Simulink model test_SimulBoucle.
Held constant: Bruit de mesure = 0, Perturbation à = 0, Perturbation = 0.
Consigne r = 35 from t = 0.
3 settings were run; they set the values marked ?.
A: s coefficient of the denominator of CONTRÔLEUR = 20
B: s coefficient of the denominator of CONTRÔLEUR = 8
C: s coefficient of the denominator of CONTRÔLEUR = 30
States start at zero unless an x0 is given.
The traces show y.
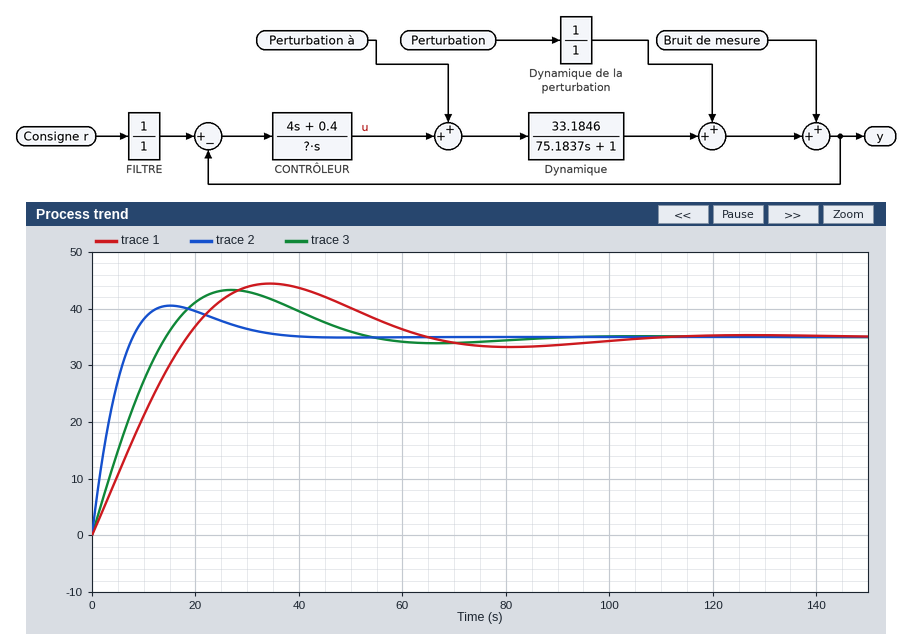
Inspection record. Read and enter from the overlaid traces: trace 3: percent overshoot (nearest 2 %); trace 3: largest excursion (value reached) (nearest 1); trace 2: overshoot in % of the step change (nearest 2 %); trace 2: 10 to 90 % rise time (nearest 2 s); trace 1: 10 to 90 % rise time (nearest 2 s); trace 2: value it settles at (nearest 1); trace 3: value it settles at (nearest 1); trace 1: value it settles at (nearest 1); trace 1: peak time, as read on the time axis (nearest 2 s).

24 %
43
16 %
6 s
14 s
35
35
35
34 s
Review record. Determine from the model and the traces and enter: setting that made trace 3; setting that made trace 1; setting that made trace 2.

A
C
B
